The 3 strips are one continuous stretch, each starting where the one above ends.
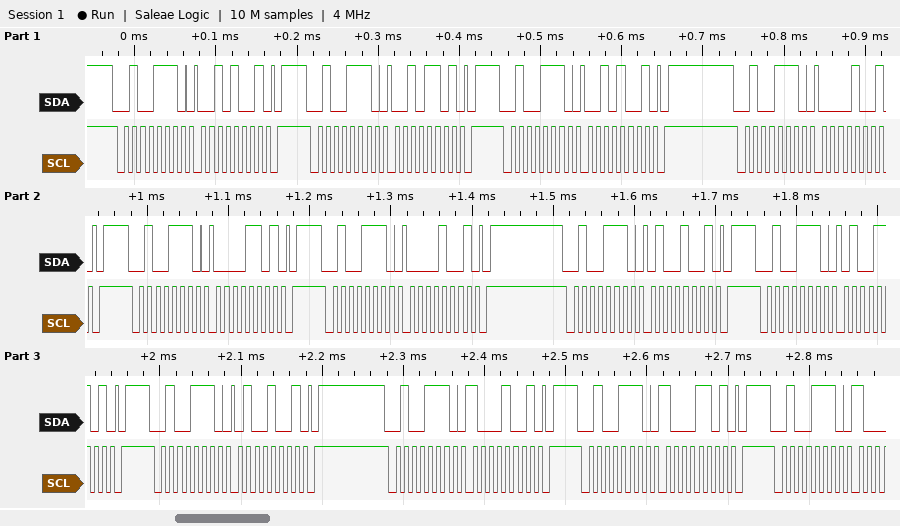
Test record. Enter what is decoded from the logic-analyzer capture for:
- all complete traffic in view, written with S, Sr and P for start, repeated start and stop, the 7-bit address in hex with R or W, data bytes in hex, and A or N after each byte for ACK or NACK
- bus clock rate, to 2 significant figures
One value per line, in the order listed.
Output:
S 27W A 29 A P S 27W A 2D A P S 27W A 29 A P S 27W A 09 A P S 27W A 0D A P S 27W A 09 A P S 27W A 49 A P S 27W A 4D A P S 27W A 49 A P S 27W A 89 A P S 27W A 8D A P S 27W A
100 kHz
